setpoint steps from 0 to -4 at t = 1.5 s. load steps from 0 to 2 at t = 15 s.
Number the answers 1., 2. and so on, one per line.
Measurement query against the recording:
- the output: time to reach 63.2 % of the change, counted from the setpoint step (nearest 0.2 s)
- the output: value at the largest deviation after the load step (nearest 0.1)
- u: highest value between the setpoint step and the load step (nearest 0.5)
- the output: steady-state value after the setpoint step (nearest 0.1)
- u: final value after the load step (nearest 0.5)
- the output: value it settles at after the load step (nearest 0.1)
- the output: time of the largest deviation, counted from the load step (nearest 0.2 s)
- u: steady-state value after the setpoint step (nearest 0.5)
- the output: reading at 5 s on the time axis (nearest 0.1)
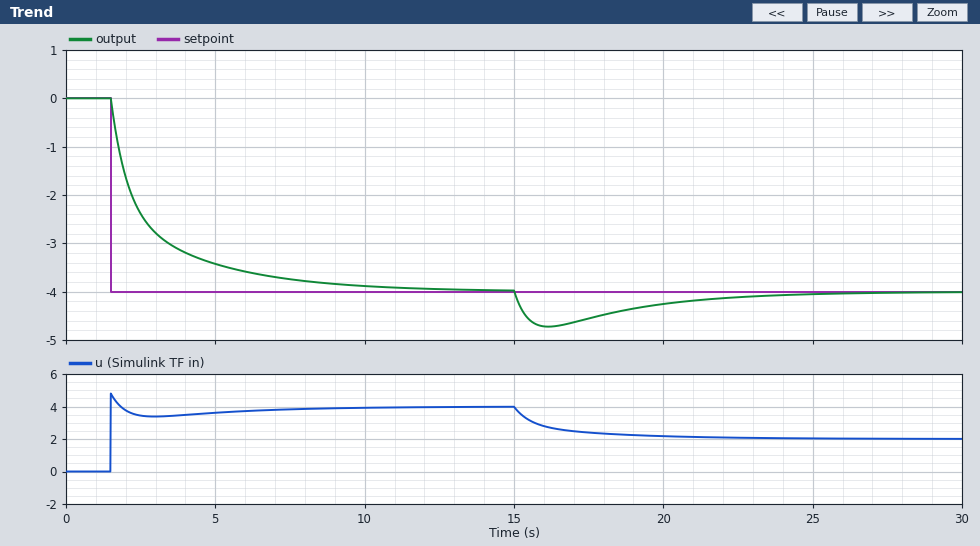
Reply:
1. 1.2 s
2. -4.7
3. 5.0
4. -4.0
5. 2.0
6. -4.0
7. 1.2 s
8. 4.0
9. -3.4
